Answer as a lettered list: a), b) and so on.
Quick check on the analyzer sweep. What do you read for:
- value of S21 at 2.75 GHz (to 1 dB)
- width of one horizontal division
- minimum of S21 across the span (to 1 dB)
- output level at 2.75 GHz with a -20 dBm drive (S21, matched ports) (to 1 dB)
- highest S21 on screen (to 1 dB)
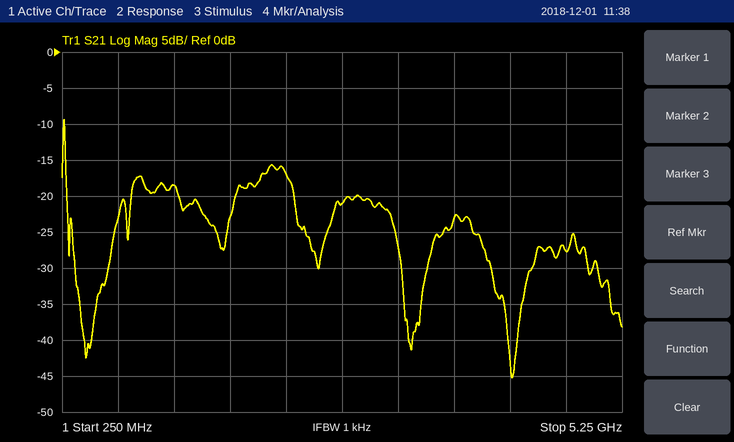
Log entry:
a) -21 dB
b) 500 MHz
c) -45 dB
d) -41 dBm
e) -9 dB
